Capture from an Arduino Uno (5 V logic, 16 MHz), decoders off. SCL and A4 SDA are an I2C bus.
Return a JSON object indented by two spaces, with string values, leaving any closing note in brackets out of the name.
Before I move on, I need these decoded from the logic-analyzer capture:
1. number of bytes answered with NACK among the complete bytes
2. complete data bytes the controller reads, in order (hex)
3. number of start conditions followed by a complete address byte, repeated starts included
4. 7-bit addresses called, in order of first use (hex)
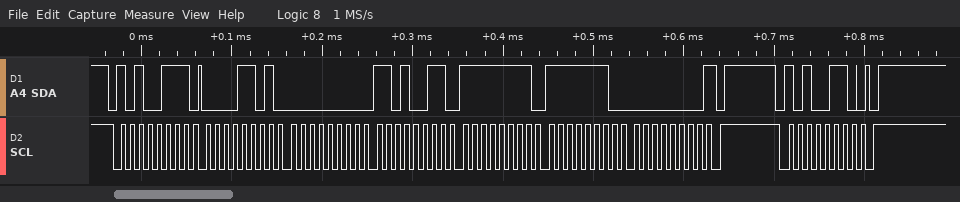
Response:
{
  "number of bytes answered with NACK among the complete bytes": "1",
  "complete data bytes the controller reads, in order": "0D 00 D3 FF FE 00",
  "number of start conditions followed by a complete address byte, repeated starts included": "2",
  "7-bit addresses called, in order of first use": "0x53"
}
